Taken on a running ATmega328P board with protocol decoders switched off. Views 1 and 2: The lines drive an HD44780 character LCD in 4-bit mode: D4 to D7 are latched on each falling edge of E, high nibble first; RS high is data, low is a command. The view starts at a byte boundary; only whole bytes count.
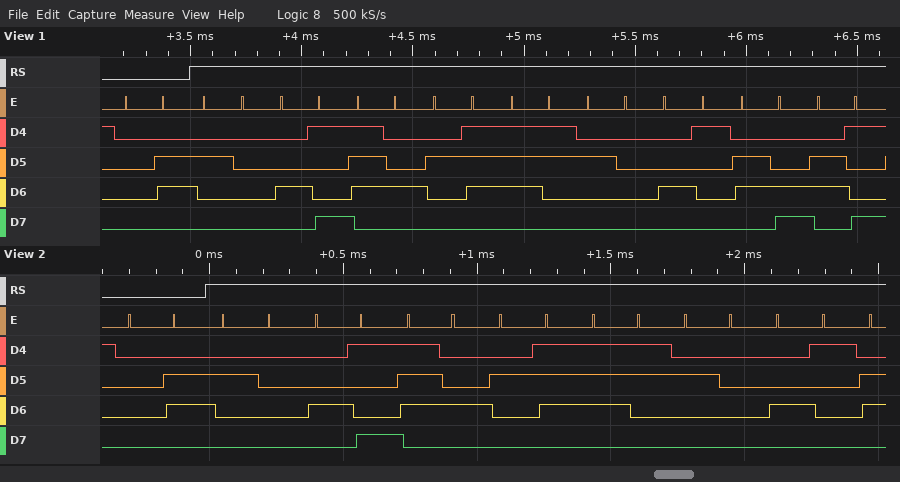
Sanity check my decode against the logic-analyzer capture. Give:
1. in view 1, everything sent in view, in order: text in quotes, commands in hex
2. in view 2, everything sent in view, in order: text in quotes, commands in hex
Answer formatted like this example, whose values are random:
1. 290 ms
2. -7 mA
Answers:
1. 0x06 " It's Ali"
2. 0x06 " It's A"
